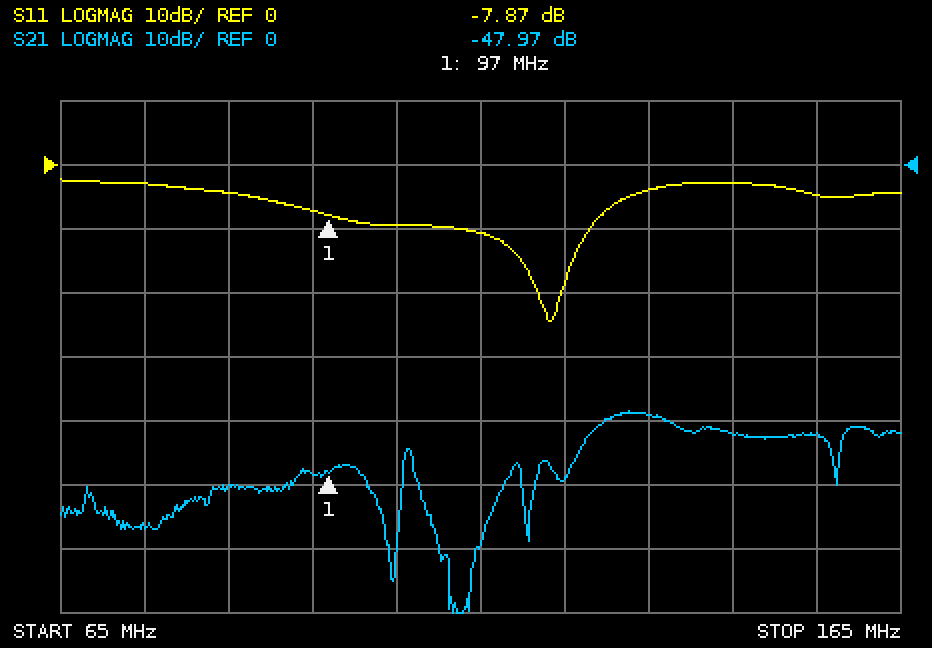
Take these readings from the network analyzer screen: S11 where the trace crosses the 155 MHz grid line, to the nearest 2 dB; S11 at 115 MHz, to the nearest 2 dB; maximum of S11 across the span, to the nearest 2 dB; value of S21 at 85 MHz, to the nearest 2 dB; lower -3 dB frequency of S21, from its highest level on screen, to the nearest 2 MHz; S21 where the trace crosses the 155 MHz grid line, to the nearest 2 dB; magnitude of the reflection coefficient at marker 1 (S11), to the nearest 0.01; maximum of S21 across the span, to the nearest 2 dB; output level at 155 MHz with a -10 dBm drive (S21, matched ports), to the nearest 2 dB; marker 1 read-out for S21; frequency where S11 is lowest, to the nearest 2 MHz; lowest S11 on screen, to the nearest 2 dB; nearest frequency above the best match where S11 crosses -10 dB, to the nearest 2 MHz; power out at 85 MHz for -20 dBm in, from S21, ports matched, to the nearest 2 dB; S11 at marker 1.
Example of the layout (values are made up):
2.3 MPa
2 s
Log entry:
-4 dB
-10 dB
-2 dB
-50 dB
128 MHz
-42 dB
0.40
-38 dB
-52 dBm
-47.97 dB
124 MHz
-24 dB
128 MHz
-70 dBm
-7.87 dB
